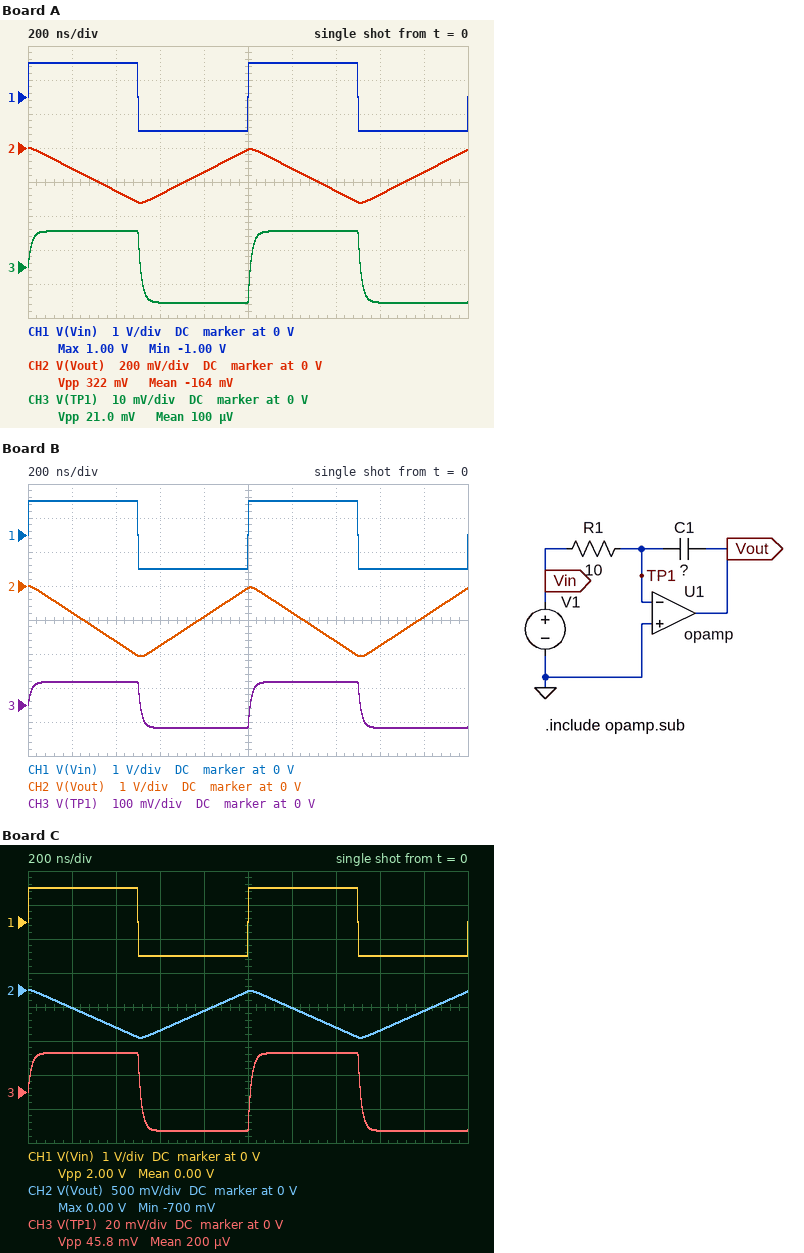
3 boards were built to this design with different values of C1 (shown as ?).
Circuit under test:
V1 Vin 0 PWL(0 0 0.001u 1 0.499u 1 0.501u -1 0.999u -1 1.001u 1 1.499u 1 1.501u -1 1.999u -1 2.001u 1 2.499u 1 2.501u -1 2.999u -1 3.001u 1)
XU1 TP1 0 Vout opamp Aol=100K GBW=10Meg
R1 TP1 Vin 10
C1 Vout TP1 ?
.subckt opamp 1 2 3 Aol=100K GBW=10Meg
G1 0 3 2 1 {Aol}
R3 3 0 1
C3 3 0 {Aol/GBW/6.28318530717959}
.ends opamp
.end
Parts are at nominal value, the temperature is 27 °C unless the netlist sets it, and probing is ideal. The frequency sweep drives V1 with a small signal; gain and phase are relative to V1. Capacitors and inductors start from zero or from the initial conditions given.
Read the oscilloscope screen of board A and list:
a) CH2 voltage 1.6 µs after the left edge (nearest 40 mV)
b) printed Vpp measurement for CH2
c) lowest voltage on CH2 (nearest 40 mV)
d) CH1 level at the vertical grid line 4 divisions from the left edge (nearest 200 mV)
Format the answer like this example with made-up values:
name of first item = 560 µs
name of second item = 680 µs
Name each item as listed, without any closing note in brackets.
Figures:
CH2 voltage 1.6 µs after the left edge = -280 mV
printed Vpp measurement for CH2 = 322 mV
lowest voltage on CH2 = -320 mV
CH1 level at the vertical grid line 4 divisions from the left edge = -1.0 V
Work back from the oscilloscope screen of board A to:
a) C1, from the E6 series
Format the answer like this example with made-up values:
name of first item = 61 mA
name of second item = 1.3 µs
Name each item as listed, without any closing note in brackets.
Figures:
C1, from the E6 series = 150 nF
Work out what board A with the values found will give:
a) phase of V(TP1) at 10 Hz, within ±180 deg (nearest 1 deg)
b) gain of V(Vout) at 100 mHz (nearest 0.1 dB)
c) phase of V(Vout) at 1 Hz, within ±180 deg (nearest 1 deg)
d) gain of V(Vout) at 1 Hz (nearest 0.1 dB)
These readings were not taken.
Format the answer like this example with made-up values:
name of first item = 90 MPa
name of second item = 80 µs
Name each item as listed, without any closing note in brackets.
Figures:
phase of V(TP1) at 10 Hz, within ±180 deg = -78 deg
gain of V(Vout) at 100 mHz = 100.0 dB
phase of V(Vout) at 1 Hz, within ±180 deg = 136 deg
gain of V(Vout) at 1 Hz = 97.2 dB
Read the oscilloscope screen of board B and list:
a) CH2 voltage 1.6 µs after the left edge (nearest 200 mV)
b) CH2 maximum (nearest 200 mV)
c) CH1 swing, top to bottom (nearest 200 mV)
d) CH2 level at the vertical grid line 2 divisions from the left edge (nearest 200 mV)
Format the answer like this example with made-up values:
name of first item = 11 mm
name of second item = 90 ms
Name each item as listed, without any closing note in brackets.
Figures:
CH2 voltage 1.6 µs after the left edge = -1.8 V
CH2 maximum = 0 V
CH1 swing, top to bottom = 2.0 V
CH2 level at the vertical grid line 2 divisions from the left edge = -1.6 V
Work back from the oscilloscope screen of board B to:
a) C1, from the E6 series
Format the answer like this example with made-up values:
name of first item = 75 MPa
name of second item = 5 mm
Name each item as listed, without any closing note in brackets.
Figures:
C1, from the E6 series = 22 nF
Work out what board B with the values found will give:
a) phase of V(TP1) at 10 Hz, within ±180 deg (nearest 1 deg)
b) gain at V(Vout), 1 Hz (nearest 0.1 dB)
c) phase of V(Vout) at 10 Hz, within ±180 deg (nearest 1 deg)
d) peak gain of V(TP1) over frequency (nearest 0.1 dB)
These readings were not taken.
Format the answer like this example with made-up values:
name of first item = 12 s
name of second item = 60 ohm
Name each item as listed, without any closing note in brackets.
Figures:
phase of V(TP1) at 10 Hz, within ±180 deg = -50 deg
gain at V(Vout), 1 Hz = 99.9 dB
phase of V(Vout) at 10 Hz, within ±180 deg = 124 deg
peak gain of V(TP1) over frequency = 0 dB
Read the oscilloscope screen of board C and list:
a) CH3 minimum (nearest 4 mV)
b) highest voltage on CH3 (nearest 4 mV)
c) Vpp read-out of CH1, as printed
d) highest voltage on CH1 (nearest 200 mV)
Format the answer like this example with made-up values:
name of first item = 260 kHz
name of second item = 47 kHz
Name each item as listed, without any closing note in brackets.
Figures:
CH3 minimum = -24 mV
highest voltage on CH3 = 24 mV
Vpp read-out of CH1, as printed = 2.00 V
highest voltage on CH1 = 1.0 V
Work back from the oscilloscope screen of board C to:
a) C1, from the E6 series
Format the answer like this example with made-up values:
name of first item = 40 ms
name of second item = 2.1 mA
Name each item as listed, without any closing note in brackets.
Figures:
C1, from the E6 series = 68 nF
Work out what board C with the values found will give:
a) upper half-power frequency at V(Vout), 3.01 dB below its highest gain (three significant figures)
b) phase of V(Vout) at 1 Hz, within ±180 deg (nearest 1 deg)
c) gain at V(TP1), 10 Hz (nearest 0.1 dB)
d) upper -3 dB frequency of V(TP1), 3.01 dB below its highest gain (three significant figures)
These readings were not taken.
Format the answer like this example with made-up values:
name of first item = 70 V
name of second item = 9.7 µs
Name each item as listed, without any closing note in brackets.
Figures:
upper half-power frequency at V(Vout), 3.01 dB below its highest gain = 2.29 Hz
phase of V(Vout) at 1 Hz, within ±180 deg = 156 deg
gain at V(TP1), 10 Hz = -13.0 dB
upper -3 dB frequency of V(TP1), 3.01 dB below its highest gain = 2.29 Hz
